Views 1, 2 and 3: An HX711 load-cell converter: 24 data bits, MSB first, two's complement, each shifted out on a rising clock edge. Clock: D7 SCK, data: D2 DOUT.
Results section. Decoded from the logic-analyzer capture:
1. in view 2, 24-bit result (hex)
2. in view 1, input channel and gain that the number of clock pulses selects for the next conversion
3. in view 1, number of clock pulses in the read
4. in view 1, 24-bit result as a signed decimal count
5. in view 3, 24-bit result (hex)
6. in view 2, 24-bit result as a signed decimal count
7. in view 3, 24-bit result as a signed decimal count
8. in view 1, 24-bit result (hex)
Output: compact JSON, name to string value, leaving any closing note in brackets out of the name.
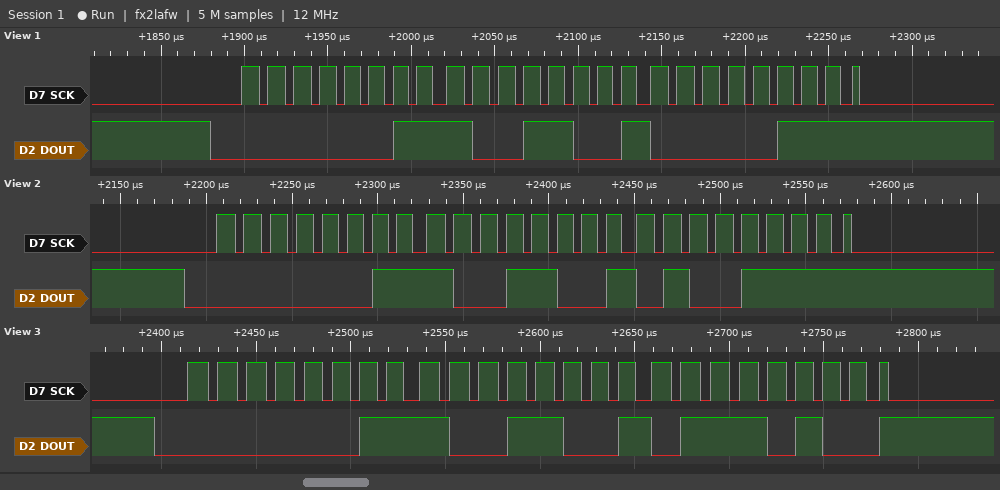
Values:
{"in view 2, 24-bit result": "0x03994F", "in view 1, input channel and gain that the number of clock pulses selects for the next conversion": "channel A, gain 128", "in view 1, number of clock pulses in the read": "25", "in view 1, 24-bit result as a signed decimal count": "235783", "in view 3, 24-bit result": "0x039974", "in view 2, 24-bit result as a signed decimal count": "235855", "in view 3, 24-bit result as a signed decimal count": "235892", "in view 1, 24-bit result": "0x039907"}
